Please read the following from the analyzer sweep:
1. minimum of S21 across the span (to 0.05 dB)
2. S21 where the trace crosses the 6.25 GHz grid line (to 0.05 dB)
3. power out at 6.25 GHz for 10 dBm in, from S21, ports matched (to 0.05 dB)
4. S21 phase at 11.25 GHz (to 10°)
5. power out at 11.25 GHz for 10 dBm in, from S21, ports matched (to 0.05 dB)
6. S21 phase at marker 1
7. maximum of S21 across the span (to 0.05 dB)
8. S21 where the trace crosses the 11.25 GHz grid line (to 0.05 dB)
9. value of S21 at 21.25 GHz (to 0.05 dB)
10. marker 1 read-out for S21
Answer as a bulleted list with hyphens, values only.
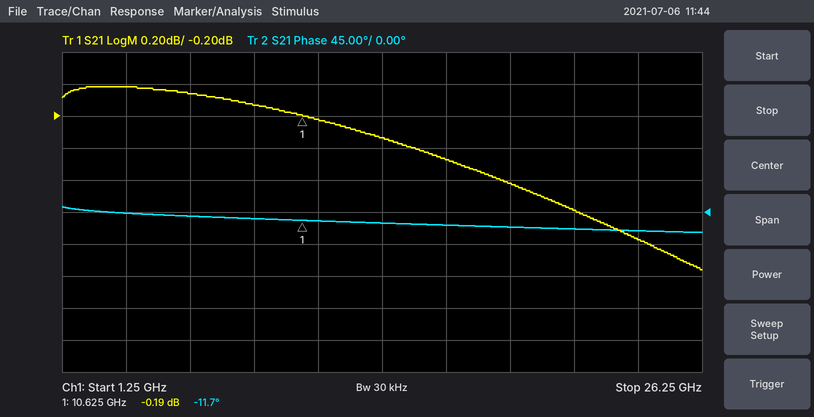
- -1.15 dB
- -0.05 dB
- 9.95 dBm
- -10°
- 9.80 dBm
- -11.7°
- 0.00 dB
- -0.20 dB
- -0.80 dB
- -0.19 dB
